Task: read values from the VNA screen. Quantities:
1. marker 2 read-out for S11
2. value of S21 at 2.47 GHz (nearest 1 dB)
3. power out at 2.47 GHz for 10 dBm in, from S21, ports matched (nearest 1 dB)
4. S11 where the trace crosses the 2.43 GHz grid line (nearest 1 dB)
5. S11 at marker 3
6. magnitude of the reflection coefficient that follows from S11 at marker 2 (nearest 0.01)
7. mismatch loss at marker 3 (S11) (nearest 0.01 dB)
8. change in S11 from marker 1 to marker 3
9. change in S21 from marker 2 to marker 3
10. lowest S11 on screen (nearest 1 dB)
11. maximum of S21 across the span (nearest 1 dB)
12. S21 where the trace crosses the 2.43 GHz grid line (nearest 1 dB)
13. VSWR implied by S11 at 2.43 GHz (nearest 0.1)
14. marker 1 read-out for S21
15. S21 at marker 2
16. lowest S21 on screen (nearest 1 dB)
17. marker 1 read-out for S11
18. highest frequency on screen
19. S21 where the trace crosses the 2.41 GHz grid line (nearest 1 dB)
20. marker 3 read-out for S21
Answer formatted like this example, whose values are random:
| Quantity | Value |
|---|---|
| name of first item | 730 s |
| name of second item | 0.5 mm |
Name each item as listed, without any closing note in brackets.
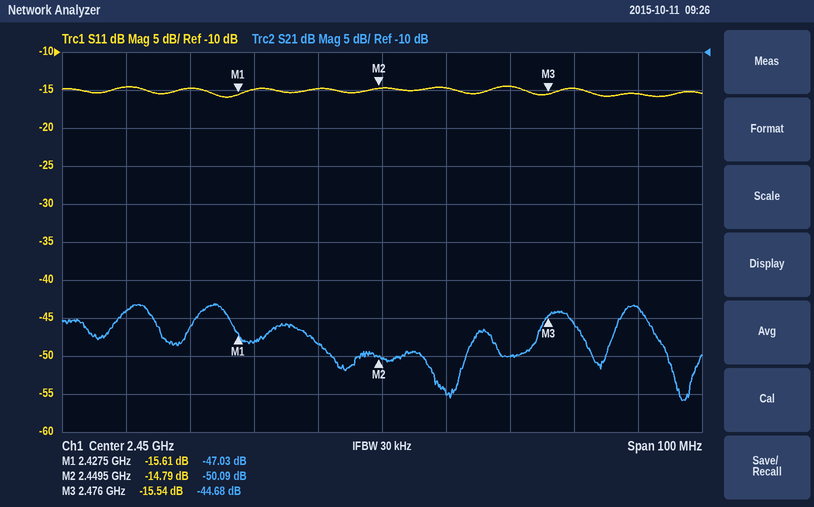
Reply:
| Quantity | Value |
|---|---|
| marker 2 read-out for S11 | -14.79 dB |
| value of S21 at 2.47 GHz | -50 dB |
| power out at 2.47 GHz for 10 dBm in, from S21, ports matched | -40 dBm |
| S11 where the trace crosses the 2.43 GHz grid line | -15 dB |
| S11 at marker 3 | -15.54 dB |
| magnitude of the reflection coefficient that follows from S11 at marker 2 | 0.18 |
| mismatch loss at marker 3 (S11) | 0.12 dB |
| change in S11 from marker 1 to marker 3 | 0.07 dB |
| change in S21 from marker 2 to marker 3 | 5.41 dB |
| lowest S11 on screen | -16 dB |
| maximum of S21 across the span | -43 dB |
| S21 where the trace crosses the 2.43 GHz grid line | -48 dB |
| VSWR implied by S11 at 2.43 GHz | 1.4 |
| marker 1 read-out for S21 | -47.03 dB |
| S21 at marker 2 | -50.09 dB |
| lowest S21 on screen | -56 dB |
| marker 1 read-out for S11 | -15.61 dB |
| highest frequency on screen | 2.5 GHz |
| S21 where the trace crosses the 2.41 GHz grid line | -44 dB |
| marker 3 read-out for S21 | -44.68 dB |
